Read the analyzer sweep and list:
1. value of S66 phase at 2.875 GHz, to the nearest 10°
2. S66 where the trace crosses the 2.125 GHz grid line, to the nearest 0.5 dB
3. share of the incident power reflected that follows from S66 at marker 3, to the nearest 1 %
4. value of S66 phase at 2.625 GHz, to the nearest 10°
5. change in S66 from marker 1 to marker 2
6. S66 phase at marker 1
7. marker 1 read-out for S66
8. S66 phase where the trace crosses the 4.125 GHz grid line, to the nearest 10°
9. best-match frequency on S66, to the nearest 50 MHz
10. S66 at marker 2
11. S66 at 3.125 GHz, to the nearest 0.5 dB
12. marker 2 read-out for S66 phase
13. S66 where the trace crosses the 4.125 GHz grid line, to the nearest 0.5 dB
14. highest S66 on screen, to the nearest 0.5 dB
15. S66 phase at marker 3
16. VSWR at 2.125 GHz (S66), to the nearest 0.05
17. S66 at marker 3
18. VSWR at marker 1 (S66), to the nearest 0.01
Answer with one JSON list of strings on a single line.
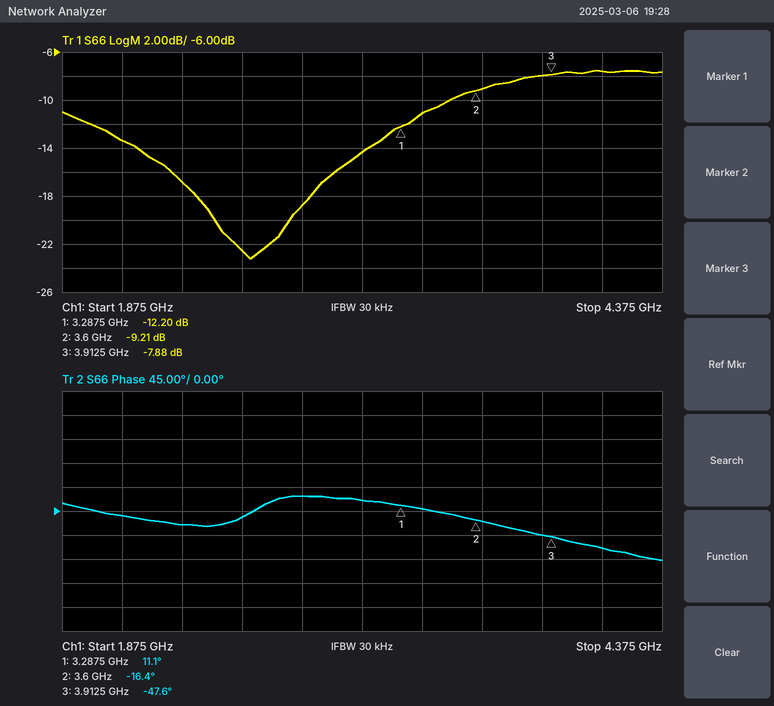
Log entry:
["30°", "-13.5 dB", "16 %", "-10°", "2.99 dB", "11.1°", "-12.20 dB", "-70°", "2.65 GHz", "-9.21 dB", "-14.5 dB", "-16.4°", "-7.5 dB", "-7.5 dB", "-47.6°", "1.55", "-7.88 dB", "1.65"]
